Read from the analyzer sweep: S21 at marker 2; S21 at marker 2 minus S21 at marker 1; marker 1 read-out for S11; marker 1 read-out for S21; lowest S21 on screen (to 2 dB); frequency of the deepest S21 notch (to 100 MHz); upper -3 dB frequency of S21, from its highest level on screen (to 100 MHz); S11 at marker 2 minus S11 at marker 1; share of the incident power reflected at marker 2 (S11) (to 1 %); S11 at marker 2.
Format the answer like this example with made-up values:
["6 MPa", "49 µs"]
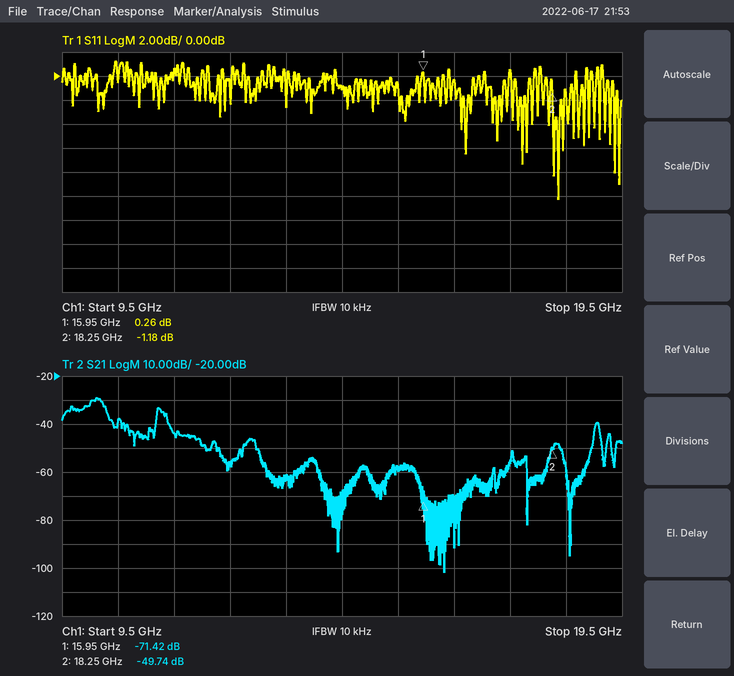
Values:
["-49.74 dB", "21.68 dB", "0.26 dB", "-71.42 dB", "-102 dB", "16.3 GHz", "10.2 GHz", "-1.44 dB", "76 %", "-1.18 dB"]
